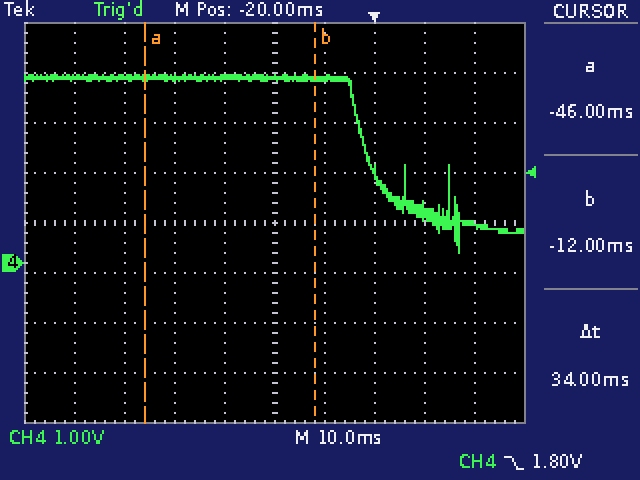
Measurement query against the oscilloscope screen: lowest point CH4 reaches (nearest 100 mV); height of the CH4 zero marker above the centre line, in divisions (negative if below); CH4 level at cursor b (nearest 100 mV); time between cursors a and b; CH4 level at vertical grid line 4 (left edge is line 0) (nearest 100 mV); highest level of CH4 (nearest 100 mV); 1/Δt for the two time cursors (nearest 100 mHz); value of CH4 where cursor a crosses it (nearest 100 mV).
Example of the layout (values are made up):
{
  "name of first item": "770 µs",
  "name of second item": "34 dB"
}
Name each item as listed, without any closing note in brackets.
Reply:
{
  "lowest point CH4 reaches": "200 mV",
  "height of the CH4 zero marker above the centre line, in divisions": "-0.8 div",
  "CH4 level at cursor b": "3.7 V",
  "time between cursors a and b": "34 ms",
  "CH4 level at vertical grid line 4 (left edge is line 0)": "3.7 V",
  "highest level of CH4": "3.8 V",
  "1/Δt for the two time cursors": "29.4 Hz",
  "value of CH4 where cursor a crosses it": "3.7 V"
}
